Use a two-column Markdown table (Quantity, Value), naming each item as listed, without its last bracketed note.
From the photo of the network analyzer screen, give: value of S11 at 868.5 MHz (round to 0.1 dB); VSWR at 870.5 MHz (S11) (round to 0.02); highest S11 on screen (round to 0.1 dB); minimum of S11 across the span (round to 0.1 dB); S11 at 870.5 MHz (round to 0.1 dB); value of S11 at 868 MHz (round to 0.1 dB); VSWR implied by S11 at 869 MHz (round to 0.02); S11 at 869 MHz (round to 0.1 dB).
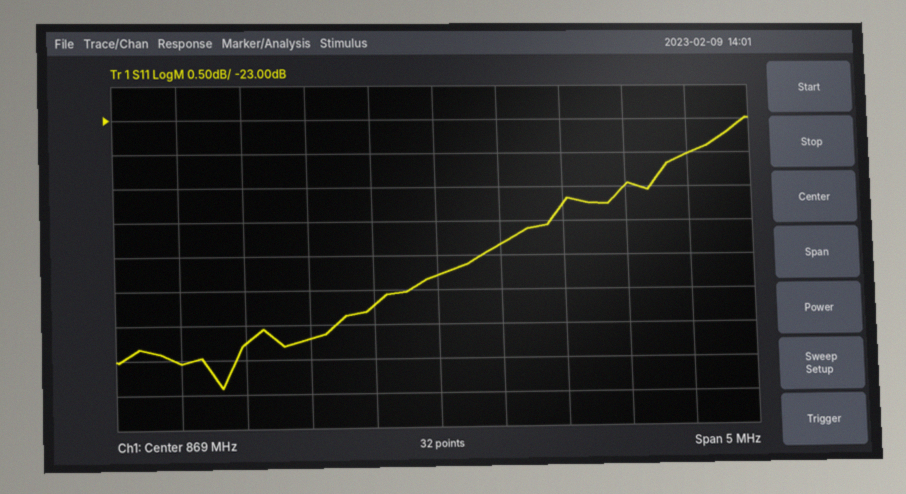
| Quantity | Value |
|---|---|
| value of S11 at 868.5 MHz | -25.7 dB |
| VSWR at 870.5 MHz (S11) | 1.14 |
| highest S11 on screen | -23.0 dB |
| minimum of S11 across the span | -26.9 dB |
| S11 at 870.5 MHz | -24.0 dB |
| value of S11 at 868 MHz | -26.2 dB |
| VSWR implied by S11 at 869 MHz | 1.12 |
| S11 at 869 MHz | -25.3 dB |
